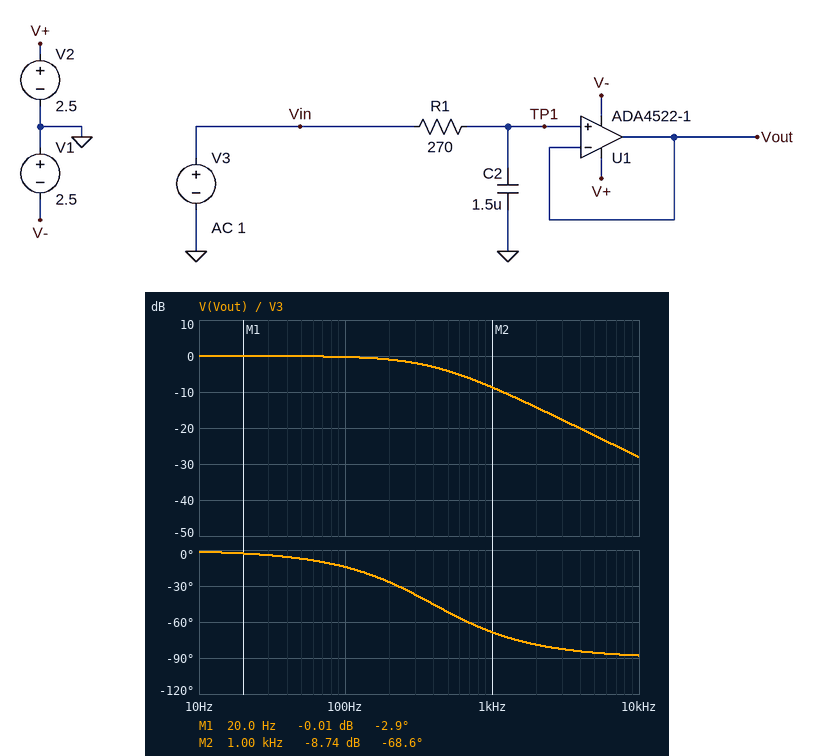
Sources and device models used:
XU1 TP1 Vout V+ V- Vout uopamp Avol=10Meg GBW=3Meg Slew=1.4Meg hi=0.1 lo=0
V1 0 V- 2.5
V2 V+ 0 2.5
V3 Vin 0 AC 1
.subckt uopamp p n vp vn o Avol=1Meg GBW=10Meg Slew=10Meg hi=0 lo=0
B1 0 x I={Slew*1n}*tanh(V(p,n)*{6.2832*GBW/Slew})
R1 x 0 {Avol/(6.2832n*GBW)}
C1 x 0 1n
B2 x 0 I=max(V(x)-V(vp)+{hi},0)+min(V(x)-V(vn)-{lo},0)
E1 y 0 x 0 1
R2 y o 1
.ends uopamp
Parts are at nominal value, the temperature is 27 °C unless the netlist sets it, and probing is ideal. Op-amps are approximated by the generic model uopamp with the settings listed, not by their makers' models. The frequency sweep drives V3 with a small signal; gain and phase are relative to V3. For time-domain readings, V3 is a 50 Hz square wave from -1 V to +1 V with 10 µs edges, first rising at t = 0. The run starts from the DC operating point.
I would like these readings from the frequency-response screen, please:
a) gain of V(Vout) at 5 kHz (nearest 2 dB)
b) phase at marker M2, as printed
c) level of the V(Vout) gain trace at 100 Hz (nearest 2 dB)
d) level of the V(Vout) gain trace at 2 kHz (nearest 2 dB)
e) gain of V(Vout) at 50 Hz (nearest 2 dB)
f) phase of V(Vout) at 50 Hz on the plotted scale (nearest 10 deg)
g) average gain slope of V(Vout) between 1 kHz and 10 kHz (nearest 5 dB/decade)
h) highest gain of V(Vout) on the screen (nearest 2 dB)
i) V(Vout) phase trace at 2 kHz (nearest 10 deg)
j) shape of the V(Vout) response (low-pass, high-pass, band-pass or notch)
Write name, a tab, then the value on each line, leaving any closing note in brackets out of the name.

gain of V(Vout) at 5 kHz	-22 dB
phase at marker M2, as printed	-68.6 deg
level of the V(Vout) gain trace at 100 Hz	0 dB
level of the V(Vout) gain trace at 2 kHz	-14 dB
gain of V(Vout) at 50 Hz	0 dB
phase of V(Vout) at 50 Hz on the plotted scale	-10 deg
average gain slope of V(Vout) between 1 kHz and 10 kHz	-20 dB/decade
highest gain of V(Vout) on the screen	0 dB
V(Vout) phase trace at 2 kHz	-80 deg
shape of the V(Vout) response	low-pass
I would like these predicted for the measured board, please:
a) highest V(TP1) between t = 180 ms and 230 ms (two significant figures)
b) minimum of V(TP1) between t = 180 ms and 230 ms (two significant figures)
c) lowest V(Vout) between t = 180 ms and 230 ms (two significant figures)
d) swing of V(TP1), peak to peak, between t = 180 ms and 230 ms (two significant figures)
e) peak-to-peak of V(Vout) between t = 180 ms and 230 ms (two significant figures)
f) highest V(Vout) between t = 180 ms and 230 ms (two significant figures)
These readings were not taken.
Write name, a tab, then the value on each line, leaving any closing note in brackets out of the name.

highest V(TP1) between t = 180 ms and 230 ms	1.0 V
minimum of V(TP1) between t = 180 ms and 230 ms	-1.0 V
lowest V(Vout) between t = 180 ms and 230 ms	-1.0 V
swing of V(TP1), peak to peak, between t = 180 ms and 230 ms	2.0 V
peak-to-peak of V(Vout) between t = 180 ms and 230 ms	2.0 V
highest V(Vout) between t = 180 ms and 230 ms	1.0 V
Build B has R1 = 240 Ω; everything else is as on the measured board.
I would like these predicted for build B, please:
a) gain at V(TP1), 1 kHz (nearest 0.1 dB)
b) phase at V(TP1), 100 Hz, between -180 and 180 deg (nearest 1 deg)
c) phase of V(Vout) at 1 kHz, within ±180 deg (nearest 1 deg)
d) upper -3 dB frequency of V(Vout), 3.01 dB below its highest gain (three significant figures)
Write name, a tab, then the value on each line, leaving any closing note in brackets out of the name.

gain at V(TP1), 1 kHz	-7.9 dB
phase at V(TP1), 100 Hz, between -180 and 180 deg	-13 deg
phase of V(Vout) at 1 kHz, within ±180 deg	-66 deg
upper -3 dB frequency of V(Vout), 3.01 dB below its highest gain	442 Hz
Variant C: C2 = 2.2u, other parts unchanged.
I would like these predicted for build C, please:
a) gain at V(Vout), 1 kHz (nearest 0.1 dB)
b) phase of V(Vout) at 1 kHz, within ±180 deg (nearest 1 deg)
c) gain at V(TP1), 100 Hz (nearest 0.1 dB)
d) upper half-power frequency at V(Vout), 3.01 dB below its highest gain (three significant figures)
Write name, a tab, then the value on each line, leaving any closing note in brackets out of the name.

gain at V(Vout), 1 kHz	-11.7 dB
phase of V(Vout) at 1 kHz, within ±180 deg	-75 deg
gain at V(TP1), 100 Hz	-0.6 dB
upper half-power frequency at V(Vout), 3.01 dB below its highest gain	268 Hz
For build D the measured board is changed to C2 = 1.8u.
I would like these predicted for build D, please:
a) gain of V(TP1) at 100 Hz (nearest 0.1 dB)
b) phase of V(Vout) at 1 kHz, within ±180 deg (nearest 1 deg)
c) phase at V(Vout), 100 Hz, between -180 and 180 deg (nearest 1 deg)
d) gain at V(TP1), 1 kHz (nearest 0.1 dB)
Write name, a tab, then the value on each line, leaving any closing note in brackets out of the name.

gain of V(TP1) at 100 Hz	-0.4 dB
phase of V(Vout) at 1 kHz, within ±180 deg	-72 deg
phase at V(Vout), 100 Hz, between -180 and 180 deg	-17 deg
gain at V(TP1), 1 kHz	-10.1 dB
